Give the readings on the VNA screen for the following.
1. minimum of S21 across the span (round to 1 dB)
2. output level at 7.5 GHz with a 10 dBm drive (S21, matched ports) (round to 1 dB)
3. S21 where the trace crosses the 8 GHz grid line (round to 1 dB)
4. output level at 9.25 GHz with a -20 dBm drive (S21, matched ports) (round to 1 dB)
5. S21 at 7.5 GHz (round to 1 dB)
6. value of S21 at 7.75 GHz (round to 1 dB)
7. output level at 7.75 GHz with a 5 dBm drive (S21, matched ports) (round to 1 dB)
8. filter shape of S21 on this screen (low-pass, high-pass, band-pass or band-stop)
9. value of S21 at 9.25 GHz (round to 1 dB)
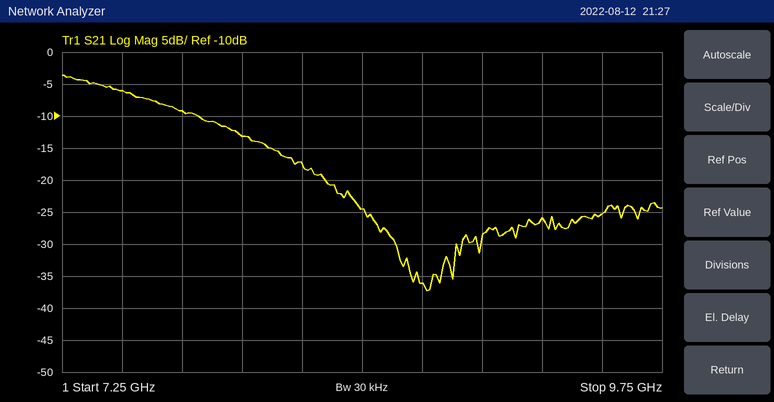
-37 dB
4 dBm
-13 dB
-46 dBm
-6 dB
-9 dB
-4 dBm
low-pass
-26 dB
